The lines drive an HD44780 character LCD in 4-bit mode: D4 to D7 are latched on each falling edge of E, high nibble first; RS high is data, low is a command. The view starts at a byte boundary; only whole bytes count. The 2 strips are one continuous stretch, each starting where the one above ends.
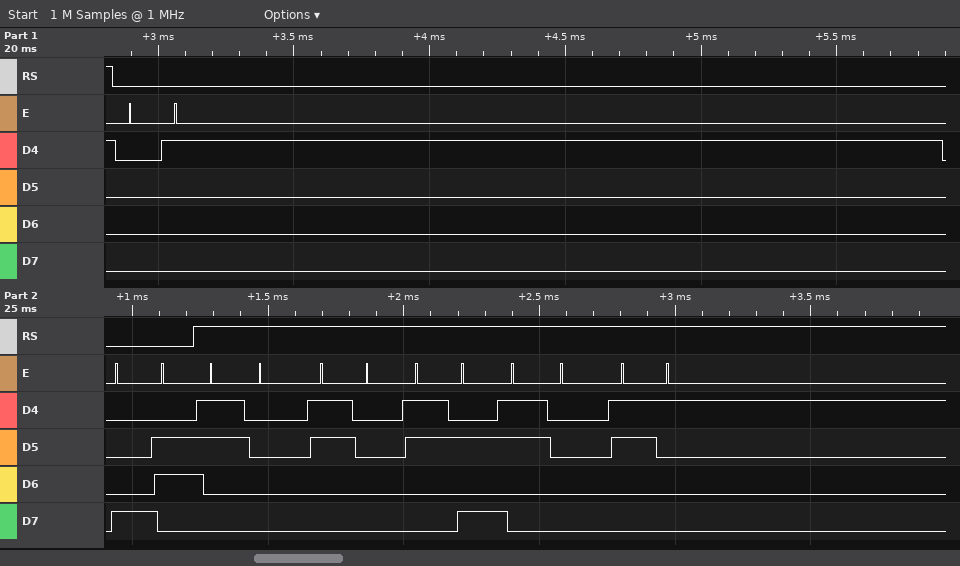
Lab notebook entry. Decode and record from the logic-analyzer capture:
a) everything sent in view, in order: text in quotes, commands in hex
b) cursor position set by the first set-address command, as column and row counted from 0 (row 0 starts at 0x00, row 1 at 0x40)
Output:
0x01 0x86 "00:01"
column 6, row 0
